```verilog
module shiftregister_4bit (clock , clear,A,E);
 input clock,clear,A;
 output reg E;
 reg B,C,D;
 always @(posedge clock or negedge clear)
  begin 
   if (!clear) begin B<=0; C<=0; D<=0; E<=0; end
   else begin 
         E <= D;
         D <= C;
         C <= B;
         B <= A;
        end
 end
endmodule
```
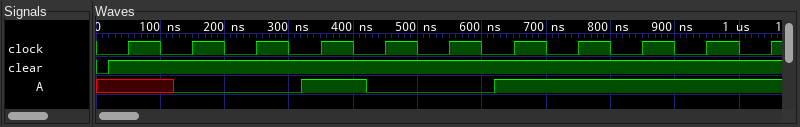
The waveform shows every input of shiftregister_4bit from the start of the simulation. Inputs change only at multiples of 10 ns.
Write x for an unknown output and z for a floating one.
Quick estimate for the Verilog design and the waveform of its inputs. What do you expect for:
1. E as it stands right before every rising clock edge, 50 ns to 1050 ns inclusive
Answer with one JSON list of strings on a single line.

["0 0 0 0 x 0 0 1 0 0 1"]
